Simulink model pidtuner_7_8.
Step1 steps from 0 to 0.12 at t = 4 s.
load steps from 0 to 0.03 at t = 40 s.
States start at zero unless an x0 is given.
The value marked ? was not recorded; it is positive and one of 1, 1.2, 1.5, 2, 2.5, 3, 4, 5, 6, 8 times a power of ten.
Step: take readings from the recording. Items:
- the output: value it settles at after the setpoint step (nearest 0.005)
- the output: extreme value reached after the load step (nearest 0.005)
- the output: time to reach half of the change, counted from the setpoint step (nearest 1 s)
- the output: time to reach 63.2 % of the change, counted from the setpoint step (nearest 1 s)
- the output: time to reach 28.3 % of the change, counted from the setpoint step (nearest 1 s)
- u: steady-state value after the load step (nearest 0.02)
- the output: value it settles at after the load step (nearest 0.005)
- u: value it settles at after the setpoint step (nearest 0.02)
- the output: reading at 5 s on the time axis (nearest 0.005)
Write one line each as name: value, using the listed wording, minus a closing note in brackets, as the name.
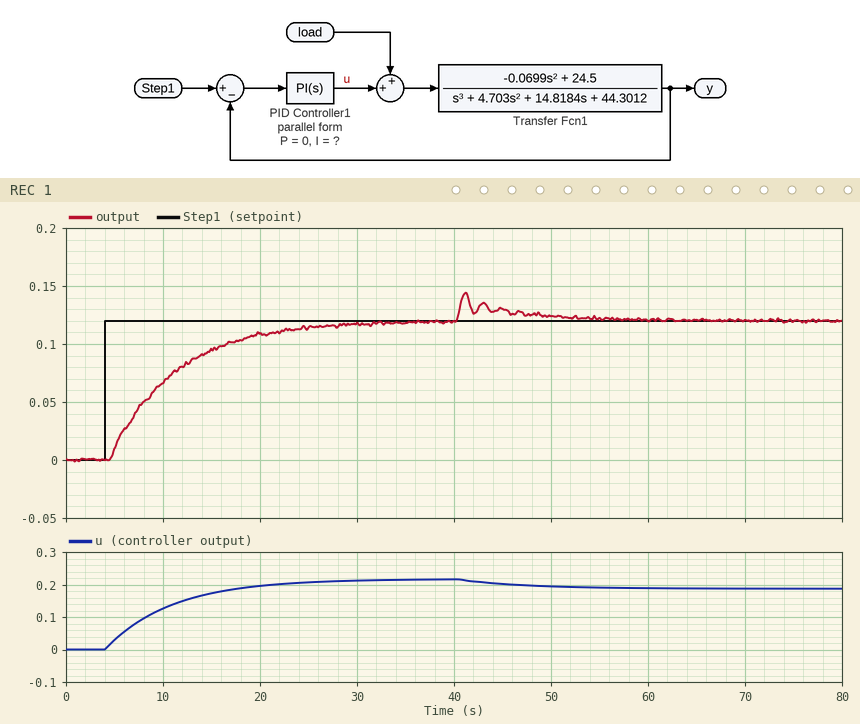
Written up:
the output: value it settles at after the setpoint step: 0.120
the output: extreme value reached after the load step: 0.145
the output: time to reach half of the change, counted from the setpoint step: 5 s
the output: time to reach 63.2 % of the change, counted from the setpoint step: 7 s
the output: time to reach 28.3 % of the change, counted from the setpoint step: 3 s
u: steady-state value after the load step: 0.18
the output: value it settles at after the load step: 0.120
u: value it settles at after the setpoint step: 0.22
the output: reading at 5 s on the time axis: 0.010
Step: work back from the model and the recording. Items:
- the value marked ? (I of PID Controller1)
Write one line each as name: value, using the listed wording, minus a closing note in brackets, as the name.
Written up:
the value marked ?: 0.25
